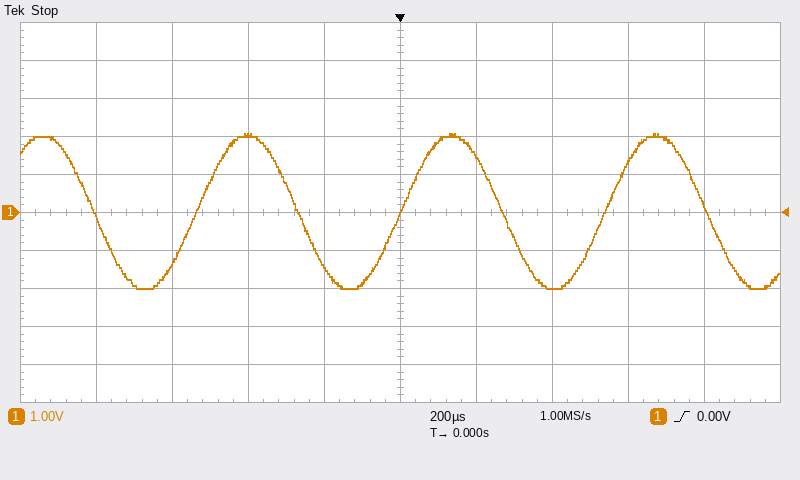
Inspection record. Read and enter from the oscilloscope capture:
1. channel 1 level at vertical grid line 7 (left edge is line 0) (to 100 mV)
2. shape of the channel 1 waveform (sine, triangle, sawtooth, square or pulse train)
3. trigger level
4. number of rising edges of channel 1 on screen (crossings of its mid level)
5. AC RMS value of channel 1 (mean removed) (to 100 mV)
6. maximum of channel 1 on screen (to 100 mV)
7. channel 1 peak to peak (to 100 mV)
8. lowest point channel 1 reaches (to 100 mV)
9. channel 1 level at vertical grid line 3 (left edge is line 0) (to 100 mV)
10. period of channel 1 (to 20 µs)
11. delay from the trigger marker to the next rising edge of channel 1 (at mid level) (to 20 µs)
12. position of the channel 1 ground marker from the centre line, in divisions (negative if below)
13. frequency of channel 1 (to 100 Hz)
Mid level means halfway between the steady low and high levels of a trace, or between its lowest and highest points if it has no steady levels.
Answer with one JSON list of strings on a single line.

["-2.0 V", "sine", "0.00 V", "3", "1.4 V", "2.1 V", "4.1 V", "-2.0 V", "2.0 V", "540 µs", "540 µs", "0.0 div", "1.9 kHz"]
